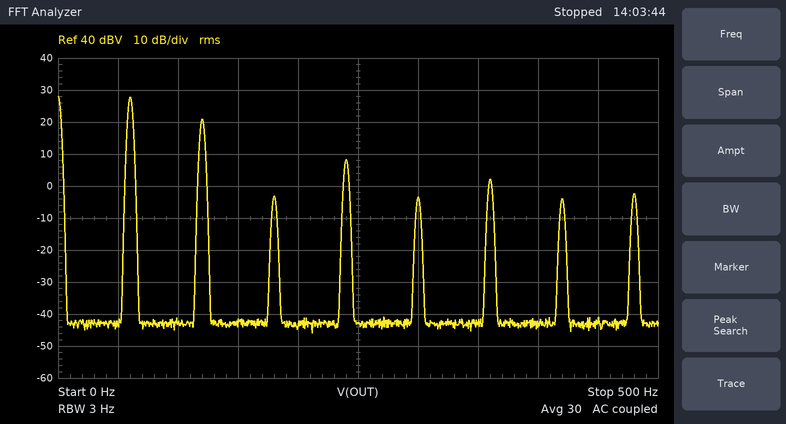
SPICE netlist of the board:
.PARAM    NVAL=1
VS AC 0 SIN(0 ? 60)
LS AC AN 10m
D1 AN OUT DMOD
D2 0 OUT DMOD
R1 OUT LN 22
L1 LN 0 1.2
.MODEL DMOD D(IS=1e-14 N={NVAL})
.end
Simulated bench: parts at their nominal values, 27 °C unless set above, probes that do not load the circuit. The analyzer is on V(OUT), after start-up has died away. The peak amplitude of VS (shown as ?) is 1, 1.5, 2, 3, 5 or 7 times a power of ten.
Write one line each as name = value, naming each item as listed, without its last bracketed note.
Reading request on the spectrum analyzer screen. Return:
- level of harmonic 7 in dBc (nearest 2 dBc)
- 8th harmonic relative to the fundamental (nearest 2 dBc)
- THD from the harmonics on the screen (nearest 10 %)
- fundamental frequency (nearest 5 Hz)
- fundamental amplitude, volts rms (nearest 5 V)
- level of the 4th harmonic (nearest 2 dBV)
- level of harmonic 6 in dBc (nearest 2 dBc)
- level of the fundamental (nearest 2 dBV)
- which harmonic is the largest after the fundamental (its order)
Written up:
level of harmonic 7 in dBc = -32 dBc
8th harmonic relative to the fundamental = -30 dBc
THD from the harmonics on the screen = 50 %
fundamental frequency = 60 Hz
fundamental amplitude, volts rms = 25 V
level of the 4th harmonic = 8 dBV
level of harmonic 6 in dBc = -26 dBc
level of the fundamental = 28 dBV
which harmonic is the largest after the fundamental = 2
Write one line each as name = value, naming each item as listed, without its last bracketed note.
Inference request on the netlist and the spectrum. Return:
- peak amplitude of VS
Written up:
peak amplitude of VS = 70 V
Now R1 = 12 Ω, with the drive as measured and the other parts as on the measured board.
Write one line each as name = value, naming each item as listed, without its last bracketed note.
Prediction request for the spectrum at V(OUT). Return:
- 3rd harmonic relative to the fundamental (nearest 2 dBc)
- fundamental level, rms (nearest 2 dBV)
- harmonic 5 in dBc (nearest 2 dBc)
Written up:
3rd harmonic relative to the fundamental = -26 dBc
fundamental level, rms = 28 dBV
harmonic 5 in dBc = -26 dBc
